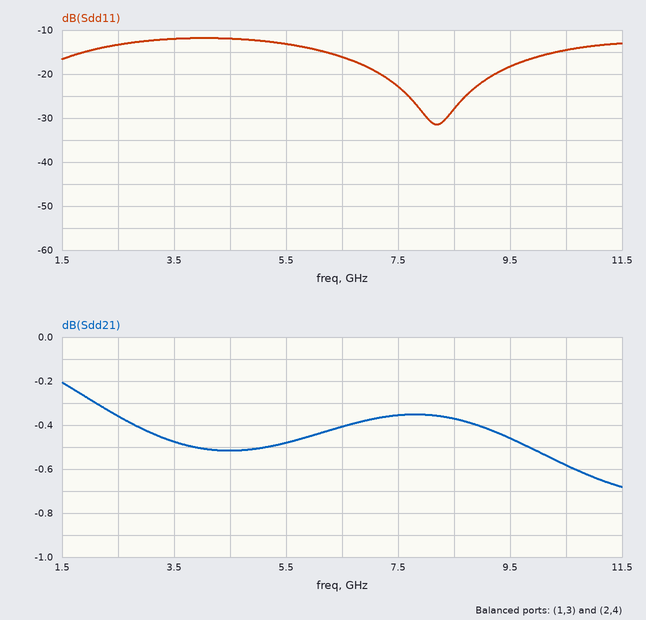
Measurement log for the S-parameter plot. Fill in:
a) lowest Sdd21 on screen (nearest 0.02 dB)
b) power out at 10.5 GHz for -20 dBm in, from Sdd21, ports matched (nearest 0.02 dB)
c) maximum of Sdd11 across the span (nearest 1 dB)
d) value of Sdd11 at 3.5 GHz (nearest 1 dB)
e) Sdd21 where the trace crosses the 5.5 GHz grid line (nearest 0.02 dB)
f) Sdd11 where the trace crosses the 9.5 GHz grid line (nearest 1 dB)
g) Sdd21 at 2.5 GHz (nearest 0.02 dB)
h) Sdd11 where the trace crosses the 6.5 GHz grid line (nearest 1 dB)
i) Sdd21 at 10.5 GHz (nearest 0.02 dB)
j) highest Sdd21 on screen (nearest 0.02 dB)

-0.68 dB
-20.58 dBm
-12 dB
-12 dB
-0.48 dB
-18 dB
-0.36 dB
-16 dB
-0.58 dB
-0.20 dB
